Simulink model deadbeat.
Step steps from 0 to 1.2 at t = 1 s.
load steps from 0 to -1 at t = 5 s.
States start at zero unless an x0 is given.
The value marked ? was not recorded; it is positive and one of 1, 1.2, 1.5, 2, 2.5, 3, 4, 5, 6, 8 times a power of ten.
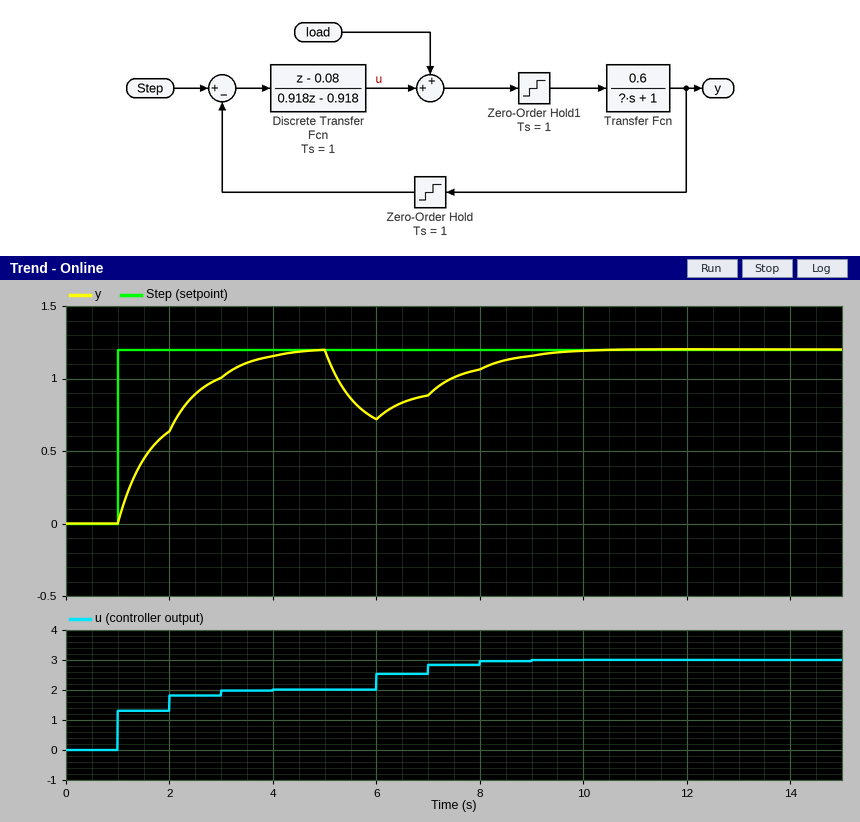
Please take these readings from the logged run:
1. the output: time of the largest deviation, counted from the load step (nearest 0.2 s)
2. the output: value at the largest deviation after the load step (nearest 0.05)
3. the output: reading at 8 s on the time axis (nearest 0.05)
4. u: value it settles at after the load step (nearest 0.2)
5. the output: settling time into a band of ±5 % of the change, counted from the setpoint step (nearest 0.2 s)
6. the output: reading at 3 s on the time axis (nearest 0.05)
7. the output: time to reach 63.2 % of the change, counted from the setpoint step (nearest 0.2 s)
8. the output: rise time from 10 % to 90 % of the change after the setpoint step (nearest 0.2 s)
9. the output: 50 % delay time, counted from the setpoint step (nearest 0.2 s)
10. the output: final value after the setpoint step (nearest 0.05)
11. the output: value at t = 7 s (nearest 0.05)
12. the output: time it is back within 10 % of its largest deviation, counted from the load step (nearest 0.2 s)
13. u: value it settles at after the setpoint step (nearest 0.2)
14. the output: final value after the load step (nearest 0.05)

1.0 s
0.70
1.05
3.0
2.8 s
1.00
1.2 s
2.2 s
0.8 s
1.20
0.90
4.0 s
2.0
1.20
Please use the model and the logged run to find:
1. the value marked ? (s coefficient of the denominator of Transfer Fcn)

0.6
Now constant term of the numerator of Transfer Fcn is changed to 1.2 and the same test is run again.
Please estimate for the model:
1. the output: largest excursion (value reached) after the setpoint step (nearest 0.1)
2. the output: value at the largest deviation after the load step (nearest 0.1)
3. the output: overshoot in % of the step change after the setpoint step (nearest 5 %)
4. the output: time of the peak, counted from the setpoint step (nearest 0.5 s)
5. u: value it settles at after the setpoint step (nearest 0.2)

1.3
0.2
10 %
2.0 s
1.0
